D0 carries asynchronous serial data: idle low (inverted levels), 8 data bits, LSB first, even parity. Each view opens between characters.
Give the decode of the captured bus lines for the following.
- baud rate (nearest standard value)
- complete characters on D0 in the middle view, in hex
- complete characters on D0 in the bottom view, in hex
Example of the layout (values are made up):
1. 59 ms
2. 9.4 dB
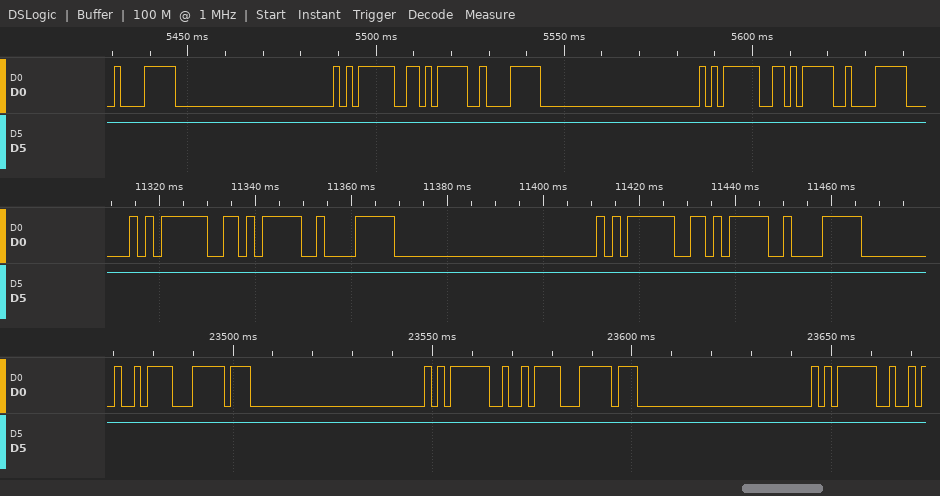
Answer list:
1. 600 baud
2. 05, 0A, 0F, 05, 0A, 0F
3. 0B, 10, 05, 0B, 10, 05
